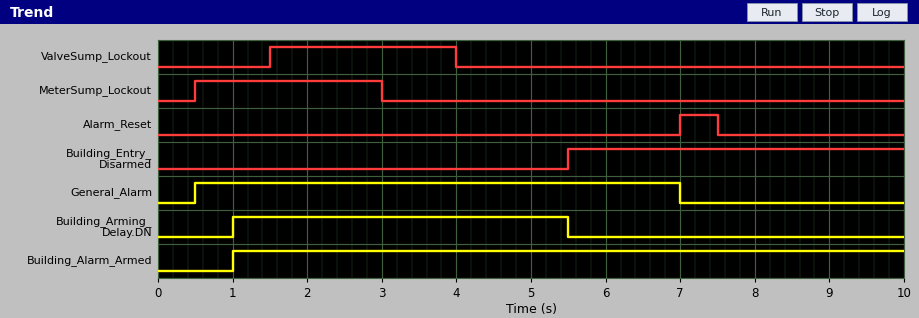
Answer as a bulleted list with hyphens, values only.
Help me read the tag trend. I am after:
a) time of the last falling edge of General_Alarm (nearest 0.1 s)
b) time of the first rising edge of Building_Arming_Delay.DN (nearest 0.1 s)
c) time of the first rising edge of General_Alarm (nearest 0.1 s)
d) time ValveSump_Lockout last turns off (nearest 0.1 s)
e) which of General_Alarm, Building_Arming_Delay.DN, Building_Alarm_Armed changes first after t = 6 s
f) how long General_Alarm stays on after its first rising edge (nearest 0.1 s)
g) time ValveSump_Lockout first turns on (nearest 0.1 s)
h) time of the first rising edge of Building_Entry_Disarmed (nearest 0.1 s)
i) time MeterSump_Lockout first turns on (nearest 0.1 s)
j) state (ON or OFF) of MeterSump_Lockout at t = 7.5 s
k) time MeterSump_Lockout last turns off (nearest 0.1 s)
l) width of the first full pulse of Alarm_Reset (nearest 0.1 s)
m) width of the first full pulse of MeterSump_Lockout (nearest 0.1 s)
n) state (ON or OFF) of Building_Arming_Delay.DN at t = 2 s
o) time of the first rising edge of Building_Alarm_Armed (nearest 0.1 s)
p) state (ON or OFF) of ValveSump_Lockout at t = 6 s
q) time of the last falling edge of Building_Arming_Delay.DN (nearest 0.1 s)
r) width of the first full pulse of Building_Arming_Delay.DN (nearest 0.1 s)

- 7.0 s
- 1.0 s
- 0.5 s
- 4.0 s
- General_Alarm
- 6.5 s
- 1.5 s
- 5.5 s
- 0.5 s
- OFF
- 3.0 s
- 0.5 s
- 2.5 s
- ON
- 1.0 s
- OFF
- 5.5 s
- 4.5 s
